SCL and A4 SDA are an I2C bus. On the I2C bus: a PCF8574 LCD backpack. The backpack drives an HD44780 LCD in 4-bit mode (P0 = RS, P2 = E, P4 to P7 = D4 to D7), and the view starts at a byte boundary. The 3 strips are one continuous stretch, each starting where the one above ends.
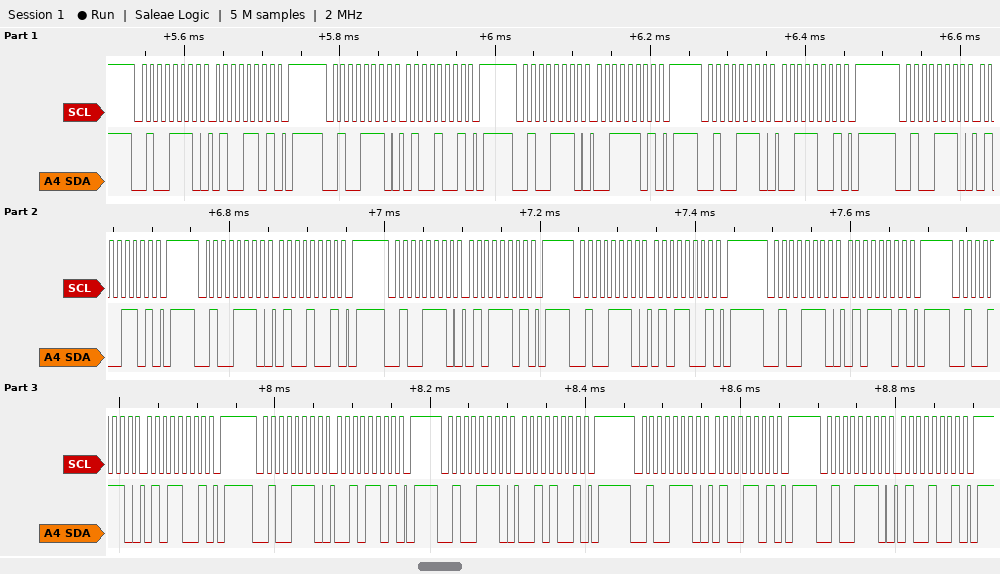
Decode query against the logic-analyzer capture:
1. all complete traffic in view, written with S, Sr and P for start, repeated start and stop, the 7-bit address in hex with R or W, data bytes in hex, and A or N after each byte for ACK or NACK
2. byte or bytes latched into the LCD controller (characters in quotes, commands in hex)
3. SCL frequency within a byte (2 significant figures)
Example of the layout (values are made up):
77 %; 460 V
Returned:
S 27W A 4D A P S 27W A 49 A P S 27W A 3D A P S 27W A 39 A P S 27W A 4D A P S 27W A 49 A P S 27W A 5D A P S 27W A 59 A P S 27W A 5D A P S 27W A 59 A P S 27W A 2D A P S 27W A 29 A P S 27W A 4D A P S 27W A 49 A P; 'C' 'E' 'R'; 100 kHz
